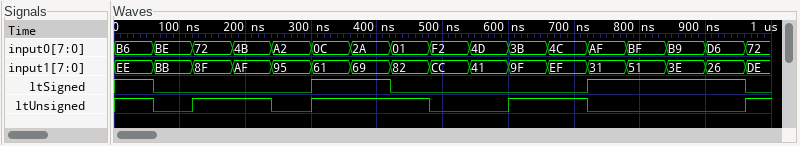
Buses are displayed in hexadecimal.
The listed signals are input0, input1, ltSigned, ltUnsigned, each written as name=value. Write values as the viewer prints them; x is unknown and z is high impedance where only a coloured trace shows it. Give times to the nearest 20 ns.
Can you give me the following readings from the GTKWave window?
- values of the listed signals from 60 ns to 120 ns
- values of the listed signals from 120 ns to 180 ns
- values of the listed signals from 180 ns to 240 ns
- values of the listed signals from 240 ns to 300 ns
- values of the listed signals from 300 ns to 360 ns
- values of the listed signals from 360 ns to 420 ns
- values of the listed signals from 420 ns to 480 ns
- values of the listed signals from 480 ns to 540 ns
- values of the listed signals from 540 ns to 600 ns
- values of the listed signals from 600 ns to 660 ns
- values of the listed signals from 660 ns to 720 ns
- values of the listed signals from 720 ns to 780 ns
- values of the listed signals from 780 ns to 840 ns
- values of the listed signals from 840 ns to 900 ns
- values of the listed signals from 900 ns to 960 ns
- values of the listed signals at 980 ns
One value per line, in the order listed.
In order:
input0=BE, input1=BB, ltSigned=0, ltUnsigned=0
input0=72, input1=8F, ltSigned=0, ltUnsigned=1
input0=4B, input1=AF, ltSigned=0, ltUnsigned=1
input0=A2, input1=95, ltSigned=0, ltUnsigned=0
input0=0C, input1=61, ltSigned=1, ltUnsigned=1
input0=2A, input1=69, ltSigned=1, ltUnsigned=1
input0=01, input1=82, ltSigned=0, ltUnsigned=1
input0=F2, input1=CC, ltSigned=0, ltUnsigned=0
input0=4D, input1=41, ltSigned=0, ltUnsigned=0
input0=3B, input1=9F, ltSigned=0, ltUnsigned=1
input0=4C, input1=EF, ltSigned=0, ltUnsigned=1
input0=AF, input1=31, ltSigned=1, ltUnsigned=0
input0=BF, input1=51, ltSigned=1, ltUnsigned=0
input0=B9, input1=3E, ltSigned=1, ltUnsigned=0
input0=D6, input1=26, ltSigned=1, ltUnsigned=0
input0=72, input1=DE, ltSigned=0, ltUnsigned=1
